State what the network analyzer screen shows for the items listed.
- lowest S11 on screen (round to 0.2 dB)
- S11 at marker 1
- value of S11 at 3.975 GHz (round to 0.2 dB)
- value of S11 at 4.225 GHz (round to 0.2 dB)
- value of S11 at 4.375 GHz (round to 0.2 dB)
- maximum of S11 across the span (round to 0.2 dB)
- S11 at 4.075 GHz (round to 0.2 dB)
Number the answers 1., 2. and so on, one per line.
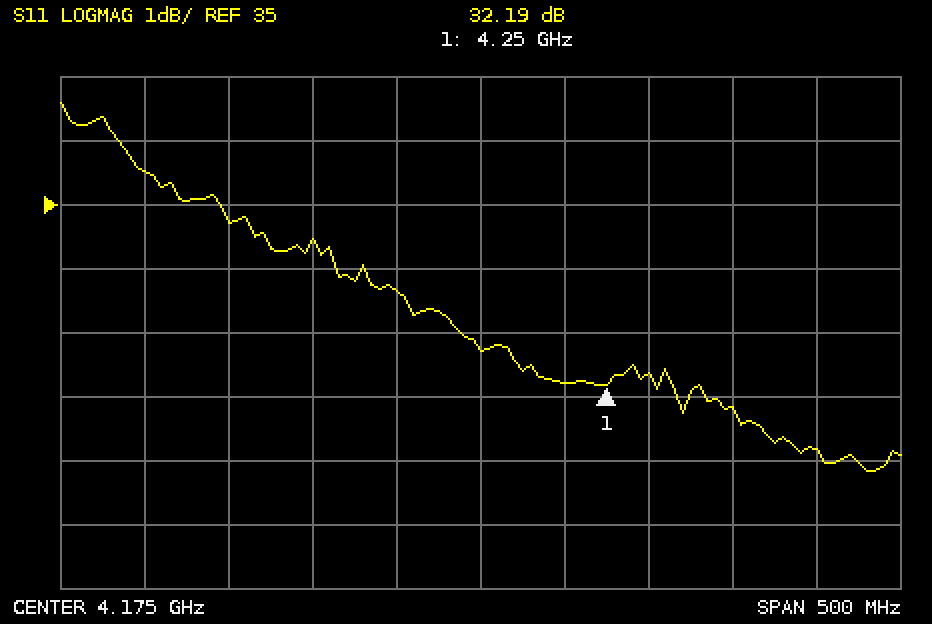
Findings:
1. 30.8 dB
2. 32.19 dB
3. 35.6 dB
4. 32.2 dB
5. 31.2 dB
6. 36.6 dB
7. 34.4 dB
